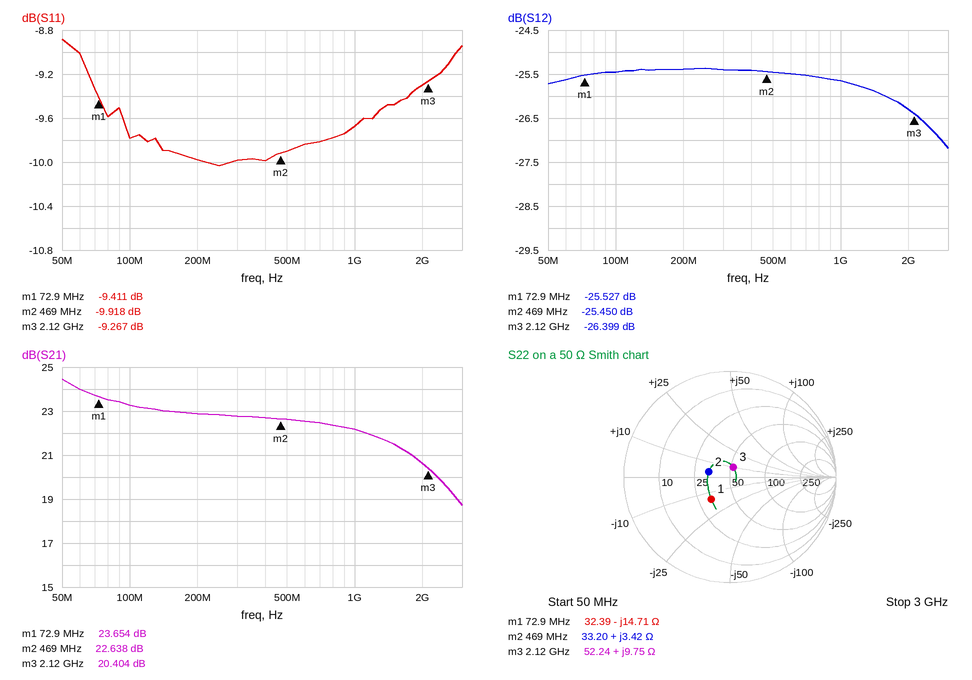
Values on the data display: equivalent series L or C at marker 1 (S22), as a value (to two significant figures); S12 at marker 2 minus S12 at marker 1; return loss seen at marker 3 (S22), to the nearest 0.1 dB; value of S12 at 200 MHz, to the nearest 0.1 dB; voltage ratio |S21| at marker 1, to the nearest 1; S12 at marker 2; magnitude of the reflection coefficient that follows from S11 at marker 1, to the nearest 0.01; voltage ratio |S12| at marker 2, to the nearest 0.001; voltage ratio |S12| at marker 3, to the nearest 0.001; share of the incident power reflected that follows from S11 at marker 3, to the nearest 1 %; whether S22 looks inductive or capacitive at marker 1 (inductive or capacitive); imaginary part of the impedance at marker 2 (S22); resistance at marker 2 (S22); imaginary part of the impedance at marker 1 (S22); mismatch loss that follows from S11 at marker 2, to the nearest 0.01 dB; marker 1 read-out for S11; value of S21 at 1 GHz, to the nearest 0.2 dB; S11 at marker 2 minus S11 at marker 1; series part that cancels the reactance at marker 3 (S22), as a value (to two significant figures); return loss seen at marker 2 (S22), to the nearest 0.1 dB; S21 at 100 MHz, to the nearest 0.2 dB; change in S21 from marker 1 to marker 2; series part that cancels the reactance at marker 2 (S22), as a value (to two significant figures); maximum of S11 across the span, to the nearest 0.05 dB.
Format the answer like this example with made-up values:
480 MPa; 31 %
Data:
150 pF; 0.077 dB; 20.2 dB; -25.4 dB; 15; -25.450 dB; 0.34; 0.053; 0.048; 12 %; capacitive; +3.42 Ω; 33.20 Ω; -14.71 Ω; 0.47 dB; -9.411 dB; 22.2 dB; -0.507 dB; 7.7 pF; 13.7 dB; 23.2 dB; -1.016 dB; 99 pF; -8.90 dB
